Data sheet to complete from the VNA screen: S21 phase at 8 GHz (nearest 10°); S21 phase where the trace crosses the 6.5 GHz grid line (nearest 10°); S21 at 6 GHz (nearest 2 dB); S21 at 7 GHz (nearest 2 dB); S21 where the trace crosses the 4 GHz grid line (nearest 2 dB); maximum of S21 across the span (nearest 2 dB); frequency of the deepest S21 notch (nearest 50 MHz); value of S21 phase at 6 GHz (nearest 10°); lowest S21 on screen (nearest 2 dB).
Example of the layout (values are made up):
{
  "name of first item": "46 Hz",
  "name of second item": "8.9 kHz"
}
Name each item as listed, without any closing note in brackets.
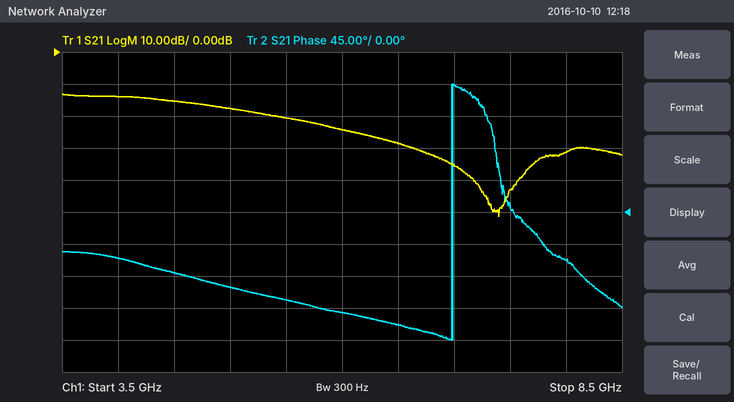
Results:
{
  "S21 phase at 8 GHz": "-70°",
  "S21 phase where the trace crosses the 6.5 GHz grid line": "-160°",
  "S21 at 6 GHz": "-24 dB",
  "S21 at 7 GHz": "-36 dB",
  "S21 where the trace crosses the 4 GHz grid line": "-14 dB",
  "maximum of S21 across the span": "-14 dB",
  "frequency of the deepest S21 notch": "7.40 GHz",
  "value of S21 phase at 6 GHz": "-140°",
  "lowest S21 on screen": "-52 dB"
}
